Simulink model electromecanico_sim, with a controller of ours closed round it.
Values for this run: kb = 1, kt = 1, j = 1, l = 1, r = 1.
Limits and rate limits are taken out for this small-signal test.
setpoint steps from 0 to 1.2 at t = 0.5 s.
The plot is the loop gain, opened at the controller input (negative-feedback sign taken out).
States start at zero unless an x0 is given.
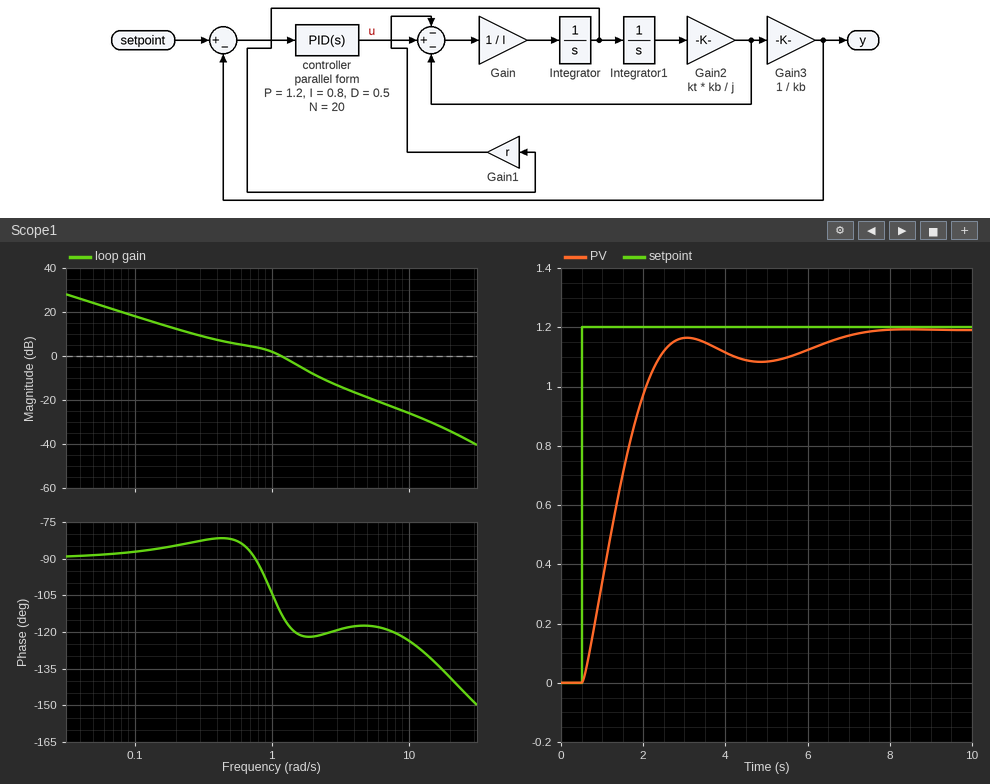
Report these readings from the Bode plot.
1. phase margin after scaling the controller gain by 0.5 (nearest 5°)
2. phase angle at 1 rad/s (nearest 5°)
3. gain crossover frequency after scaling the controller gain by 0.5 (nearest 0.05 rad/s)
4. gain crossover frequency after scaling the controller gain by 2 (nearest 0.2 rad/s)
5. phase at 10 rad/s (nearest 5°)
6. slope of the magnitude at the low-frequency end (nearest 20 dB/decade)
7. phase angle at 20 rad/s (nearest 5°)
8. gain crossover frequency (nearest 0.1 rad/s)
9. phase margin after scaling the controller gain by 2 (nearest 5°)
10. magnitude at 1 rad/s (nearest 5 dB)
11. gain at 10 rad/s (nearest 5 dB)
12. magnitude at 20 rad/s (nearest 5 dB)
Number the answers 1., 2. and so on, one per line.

1. 100°
2. -105°
3. 0.50 rad/s
4. 1.8 rad/s
5. -125°
6. -20 dB/decade
7. -140°
8. 1.2 rad/s
9. 60°
10. 0 dB
11. -25 dB
12. -35 dB
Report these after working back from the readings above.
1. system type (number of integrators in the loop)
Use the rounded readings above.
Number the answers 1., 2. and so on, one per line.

1. 1
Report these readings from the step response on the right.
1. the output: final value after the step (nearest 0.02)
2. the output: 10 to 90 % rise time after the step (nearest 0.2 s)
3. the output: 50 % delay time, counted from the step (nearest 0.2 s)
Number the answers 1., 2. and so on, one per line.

1. 1.20
2. 1.6 s
3. 0.8 s
